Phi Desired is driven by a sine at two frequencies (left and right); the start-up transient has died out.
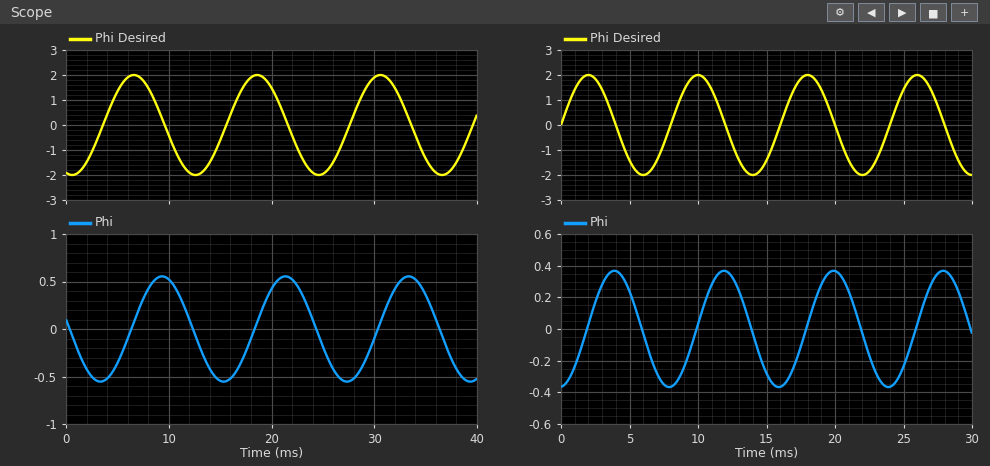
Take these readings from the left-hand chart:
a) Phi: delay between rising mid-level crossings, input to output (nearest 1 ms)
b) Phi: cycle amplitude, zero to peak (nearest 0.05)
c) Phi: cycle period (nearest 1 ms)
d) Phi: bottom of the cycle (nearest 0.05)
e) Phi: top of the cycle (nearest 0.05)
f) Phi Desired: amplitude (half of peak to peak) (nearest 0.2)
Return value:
3 ms
0.55
12 ms
-0.55
0.55
2.0
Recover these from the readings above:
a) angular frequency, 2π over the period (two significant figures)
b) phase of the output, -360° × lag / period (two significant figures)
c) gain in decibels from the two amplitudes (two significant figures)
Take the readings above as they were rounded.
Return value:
0.52 rad/ms
-90°
-11 dB
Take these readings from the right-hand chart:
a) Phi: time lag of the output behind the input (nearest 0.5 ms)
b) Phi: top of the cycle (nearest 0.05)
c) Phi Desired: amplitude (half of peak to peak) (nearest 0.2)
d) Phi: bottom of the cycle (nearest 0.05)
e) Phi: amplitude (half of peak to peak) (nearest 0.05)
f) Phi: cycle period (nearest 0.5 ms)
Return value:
2.0 ms
0.35
2.0
-0.35
0.35
8.0 ms
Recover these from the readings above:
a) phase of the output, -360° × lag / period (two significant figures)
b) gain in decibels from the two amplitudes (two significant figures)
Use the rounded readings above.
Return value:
-90°
-15 dB
